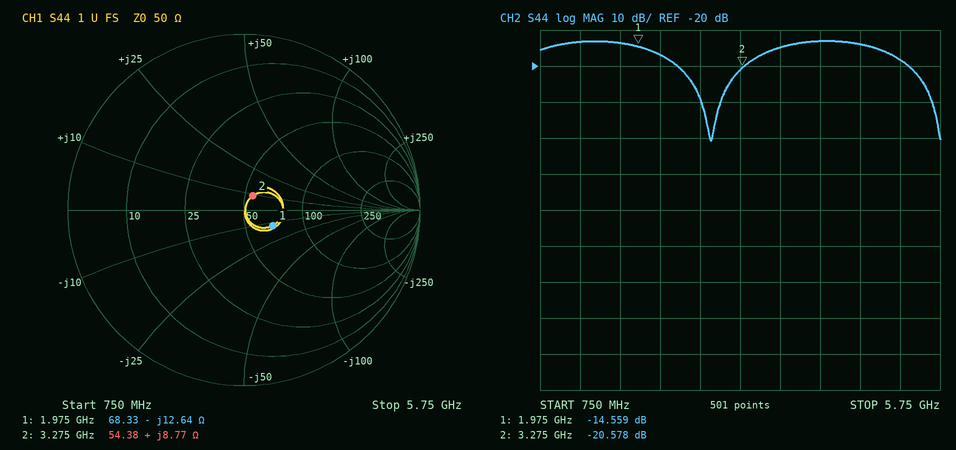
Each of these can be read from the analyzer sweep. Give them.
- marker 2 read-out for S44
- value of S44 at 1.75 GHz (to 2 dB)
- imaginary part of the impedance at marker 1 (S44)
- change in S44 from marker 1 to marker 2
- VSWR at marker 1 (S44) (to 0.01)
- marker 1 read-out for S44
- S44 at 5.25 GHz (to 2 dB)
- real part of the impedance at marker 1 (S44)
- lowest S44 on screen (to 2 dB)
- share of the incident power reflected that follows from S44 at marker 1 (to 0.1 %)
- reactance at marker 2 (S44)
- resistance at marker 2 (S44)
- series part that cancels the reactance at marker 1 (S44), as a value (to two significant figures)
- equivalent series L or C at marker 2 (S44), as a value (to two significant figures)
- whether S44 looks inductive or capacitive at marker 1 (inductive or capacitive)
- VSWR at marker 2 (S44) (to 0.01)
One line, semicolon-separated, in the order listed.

-20.578 dB; -14 dB; -12.64 Ω; -6.019 dB; 1.46; -14.559 dB; -18 dB; 68.33 Ω; -40 dB; 3.5 %; +8.77 Ω; 54.38 Ω; 1.0 nH; 430 pH; capacitive; 1.21
